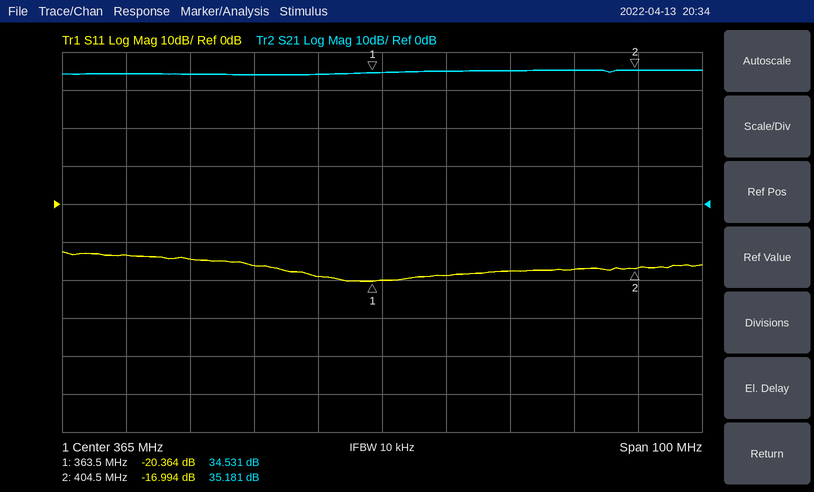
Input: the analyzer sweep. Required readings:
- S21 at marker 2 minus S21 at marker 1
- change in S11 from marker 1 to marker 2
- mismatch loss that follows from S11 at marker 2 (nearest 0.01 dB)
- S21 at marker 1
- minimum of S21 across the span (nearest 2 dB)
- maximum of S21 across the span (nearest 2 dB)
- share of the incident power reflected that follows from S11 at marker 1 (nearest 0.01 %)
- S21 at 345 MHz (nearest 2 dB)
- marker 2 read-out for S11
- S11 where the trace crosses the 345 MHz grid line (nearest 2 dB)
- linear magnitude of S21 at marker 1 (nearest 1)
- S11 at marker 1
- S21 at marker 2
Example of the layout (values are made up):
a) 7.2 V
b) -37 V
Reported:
a) 0.650 dB
b) 3.370 dB
c) 0.09 dB
d) 34.531 dB
e) 34 dB
f) 36 dB
g) 0.92 %
h) 34 dB
i) -16.994 dB
j) -16 dB
k) 53
l) -20.364 dB
m) 35.181 dB
